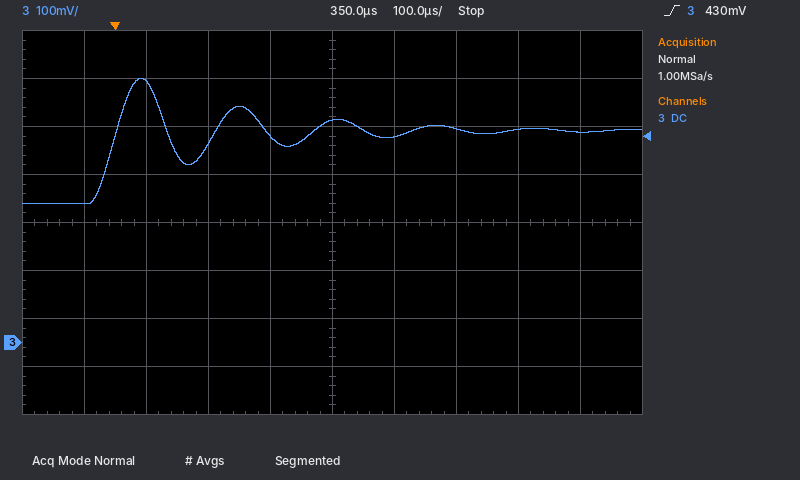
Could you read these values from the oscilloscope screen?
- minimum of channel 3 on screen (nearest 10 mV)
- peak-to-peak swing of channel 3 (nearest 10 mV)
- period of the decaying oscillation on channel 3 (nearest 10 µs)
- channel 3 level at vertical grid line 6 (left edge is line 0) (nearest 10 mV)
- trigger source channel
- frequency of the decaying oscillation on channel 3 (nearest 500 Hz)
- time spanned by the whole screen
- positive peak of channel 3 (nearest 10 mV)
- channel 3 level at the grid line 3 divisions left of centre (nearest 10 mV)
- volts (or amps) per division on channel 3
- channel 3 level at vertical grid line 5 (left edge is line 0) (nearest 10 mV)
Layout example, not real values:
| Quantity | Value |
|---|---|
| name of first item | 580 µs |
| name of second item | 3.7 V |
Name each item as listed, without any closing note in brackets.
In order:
| Quantity | Value |
|---|---|
| minimum of channel 3 on screen | 290 mV |
| peak-to-peak swing of channel 3 | 260 mV |
| period of the decaying oscillation on channel 3 | 160 µs |
| channel 3 level at vertical grid line 6 (left edge is line 0) | 430 mV |
| trigger source channel | channel 3 |
| frequency of the decaying oscillation on channel 3 | 6.5 kHz |
| time spanned by the whole screen | 1 ms |
| positive peak of channel 3 | 550 mV |
| channel 3 level at the grid line 3 divisions left of centre | 540 mV |
| volts (or amps) per division on channel 3 | 100 mV |
| channel 3 level at vertical grid line 5 (left edge is line 0) | 460 mV |
